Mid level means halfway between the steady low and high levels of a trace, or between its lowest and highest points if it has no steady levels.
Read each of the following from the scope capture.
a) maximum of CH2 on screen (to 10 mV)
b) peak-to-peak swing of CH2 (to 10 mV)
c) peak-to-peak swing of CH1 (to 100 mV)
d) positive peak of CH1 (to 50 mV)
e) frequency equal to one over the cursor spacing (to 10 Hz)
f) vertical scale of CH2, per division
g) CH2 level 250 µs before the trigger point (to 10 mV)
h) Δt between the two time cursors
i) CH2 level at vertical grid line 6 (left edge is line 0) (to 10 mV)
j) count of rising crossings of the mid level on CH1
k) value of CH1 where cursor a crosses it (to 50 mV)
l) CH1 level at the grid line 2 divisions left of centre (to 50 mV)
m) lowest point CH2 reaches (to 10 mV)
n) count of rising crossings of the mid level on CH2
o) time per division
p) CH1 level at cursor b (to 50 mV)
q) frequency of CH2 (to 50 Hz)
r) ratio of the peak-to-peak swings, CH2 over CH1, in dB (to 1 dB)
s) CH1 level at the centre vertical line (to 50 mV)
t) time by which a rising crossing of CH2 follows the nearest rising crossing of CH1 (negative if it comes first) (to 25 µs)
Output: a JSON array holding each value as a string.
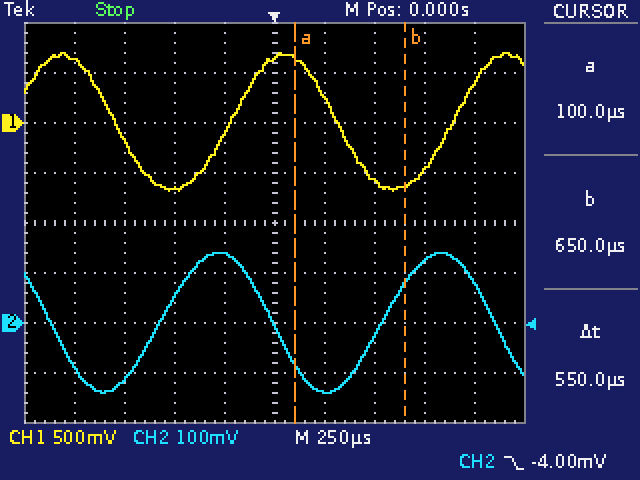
["140 mV", "280 mV", "1.40 V", "700 mV", "1.82 kHz", "100 mV", "140 mV", "550 µs", "-140 mV", "2", "650 mV", "-650 mV", "-140 mV", "2", "250 µs", "-600 mV", "900 Hz", "-14 dB", "650 mV", "-350 µs"]
